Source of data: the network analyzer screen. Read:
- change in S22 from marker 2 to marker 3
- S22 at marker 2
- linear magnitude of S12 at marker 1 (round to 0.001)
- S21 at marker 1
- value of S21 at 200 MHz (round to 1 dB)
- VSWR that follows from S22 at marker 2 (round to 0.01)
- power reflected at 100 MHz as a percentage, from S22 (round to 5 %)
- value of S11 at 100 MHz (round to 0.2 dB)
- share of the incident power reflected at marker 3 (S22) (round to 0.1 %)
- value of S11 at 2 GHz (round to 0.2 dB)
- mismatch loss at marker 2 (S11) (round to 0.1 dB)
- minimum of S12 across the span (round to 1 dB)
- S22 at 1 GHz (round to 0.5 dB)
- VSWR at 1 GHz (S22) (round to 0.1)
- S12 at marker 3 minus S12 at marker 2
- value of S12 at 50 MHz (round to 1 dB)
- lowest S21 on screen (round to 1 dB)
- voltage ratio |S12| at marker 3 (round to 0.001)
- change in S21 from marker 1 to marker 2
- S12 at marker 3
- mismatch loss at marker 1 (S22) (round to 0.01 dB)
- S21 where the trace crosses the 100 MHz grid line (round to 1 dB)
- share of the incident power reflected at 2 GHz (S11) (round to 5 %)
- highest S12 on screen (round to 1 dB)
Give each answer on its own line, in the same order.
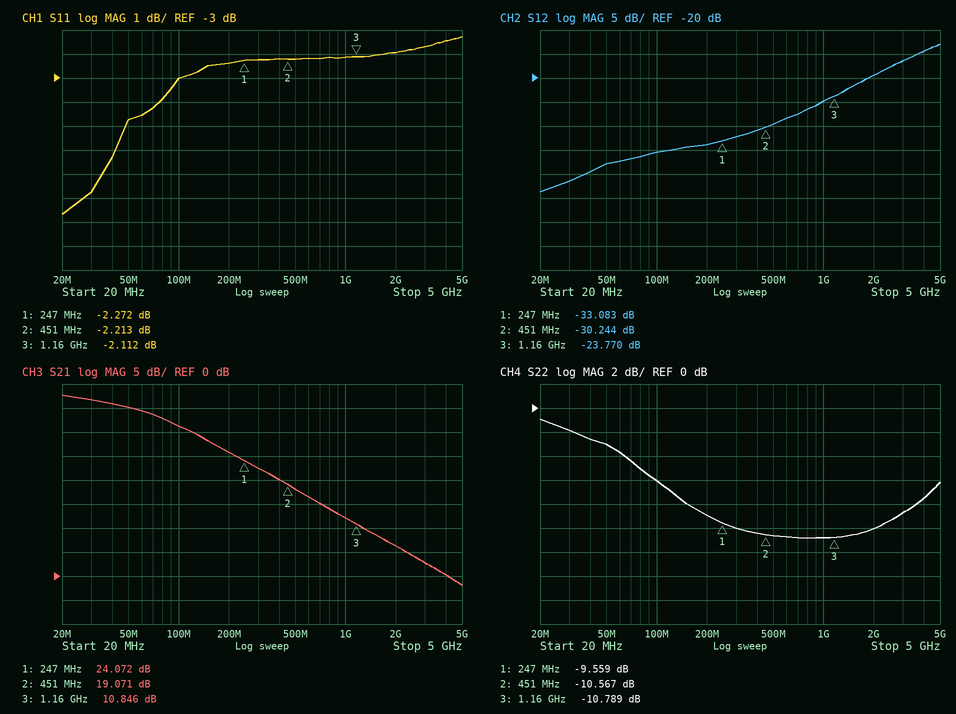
-0.222 dB
-10.567 dB
0.022
24.072 dB
26 dB
1.84
25 %
-3.0 dB
8.3 %
-2.0 dB
4.0 dB
-44 dB
-11.0 dB
1.8
6.474 dB
-38 dB
-2 dB
0.065
-5.001 dB
-23.770 dB
0.51 dB
31 dB
65 %
-13 dB
